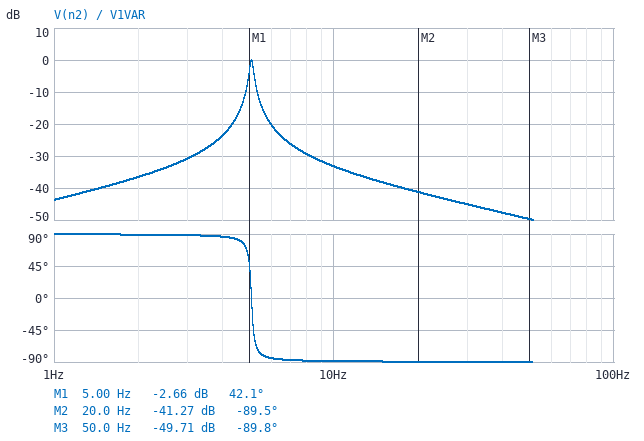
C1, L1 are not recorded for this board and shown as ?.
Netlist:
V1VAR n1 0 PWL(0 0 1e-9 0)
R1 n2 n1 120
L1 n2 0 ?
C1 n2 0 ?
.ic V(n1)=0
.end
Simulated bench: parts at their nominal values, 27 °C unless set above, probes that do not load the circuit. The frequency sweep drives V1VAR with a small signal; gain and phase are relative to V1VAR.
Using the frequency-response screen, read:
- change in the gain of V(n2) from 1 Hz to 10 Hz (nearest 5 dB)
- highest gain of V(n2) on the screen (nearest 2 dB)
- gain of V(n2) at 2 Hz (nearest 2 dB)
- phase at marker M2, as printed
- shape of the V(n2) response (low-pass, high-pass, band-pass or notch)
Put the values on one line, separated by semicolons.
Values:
10 dB; 0 dB; -36 dB; -89.5 deg; band-pass
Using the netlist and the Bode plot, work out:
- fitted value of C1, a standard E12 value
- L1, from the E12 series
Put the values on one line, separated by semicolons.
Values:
8.2 mF; 120 mH
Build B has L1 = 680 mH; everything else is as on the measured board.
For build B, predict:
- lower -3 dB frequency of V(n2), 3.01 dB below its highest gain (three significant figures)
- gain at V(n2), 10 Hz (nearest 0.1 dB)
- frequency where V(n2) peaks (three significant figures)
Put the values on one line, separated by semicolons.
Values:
2.05 Hz; -35.4 dB; 2.13 Hz
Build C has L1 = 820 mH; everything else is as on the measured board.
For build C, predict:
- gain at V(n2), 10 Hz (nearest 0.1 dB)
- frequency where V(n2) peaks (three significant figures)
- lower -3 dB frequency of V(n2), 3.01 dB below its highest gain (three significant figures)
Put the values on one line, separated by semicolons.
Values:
-35.5 dB; 1.94 Hz; 1.86 Hz
